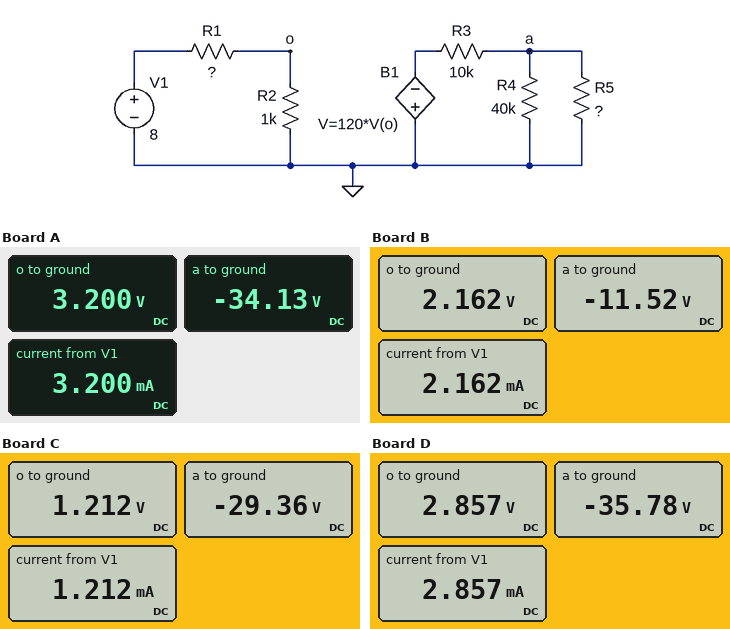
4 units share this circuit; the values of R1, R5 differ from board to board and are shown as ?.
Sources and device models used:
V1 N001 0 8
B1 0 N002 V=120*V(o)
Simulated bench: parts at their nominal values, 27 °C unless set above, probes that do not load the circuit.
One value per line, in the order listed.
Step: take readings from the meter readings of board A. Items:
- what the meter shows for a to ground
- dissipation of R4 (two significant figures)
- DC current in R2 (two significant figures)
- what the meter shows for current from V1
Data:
-34.13 V
29 mW
3.2 mA
3.200 mA
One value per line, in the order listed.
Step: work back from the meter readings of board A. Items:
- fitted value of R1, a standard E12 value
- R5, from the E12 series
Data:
1.5 kΩ
1 kΩ
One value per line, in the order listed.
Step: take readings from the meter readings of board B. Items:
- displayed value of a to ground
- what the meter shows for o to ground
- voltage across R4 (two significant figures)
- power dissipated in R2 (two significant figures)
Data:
-11.52 V
2.162 V
12 V
4.7 mW
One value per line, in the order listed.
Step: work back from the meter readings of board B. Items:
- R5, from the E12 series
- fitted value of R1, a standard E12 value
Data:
470 Ω
2.7 kΩ
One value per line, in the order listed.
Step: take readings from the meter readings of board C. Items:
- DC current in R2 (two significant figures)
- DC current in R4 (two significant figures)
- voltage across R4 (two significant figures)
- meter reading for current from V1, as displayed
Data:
1.2 mA
730 µA
29 V
1.212 mA
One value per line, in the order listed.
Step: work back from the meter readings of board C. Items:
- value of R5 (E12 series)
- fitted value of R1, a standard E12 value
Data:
2.7 kΩ
5.6 kΩ
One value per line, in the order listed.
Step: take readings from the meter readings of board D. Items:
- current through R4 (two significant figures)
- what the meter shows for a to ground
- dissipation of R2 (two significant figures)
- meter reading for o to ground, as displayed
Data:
890 µA
-35.78 V
8.2 mW
2.857 V
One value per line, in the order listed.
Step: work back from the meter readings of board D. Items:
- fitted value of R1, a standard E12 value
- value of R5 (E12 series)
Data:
1.8 kΩ
1.2 kΩ
